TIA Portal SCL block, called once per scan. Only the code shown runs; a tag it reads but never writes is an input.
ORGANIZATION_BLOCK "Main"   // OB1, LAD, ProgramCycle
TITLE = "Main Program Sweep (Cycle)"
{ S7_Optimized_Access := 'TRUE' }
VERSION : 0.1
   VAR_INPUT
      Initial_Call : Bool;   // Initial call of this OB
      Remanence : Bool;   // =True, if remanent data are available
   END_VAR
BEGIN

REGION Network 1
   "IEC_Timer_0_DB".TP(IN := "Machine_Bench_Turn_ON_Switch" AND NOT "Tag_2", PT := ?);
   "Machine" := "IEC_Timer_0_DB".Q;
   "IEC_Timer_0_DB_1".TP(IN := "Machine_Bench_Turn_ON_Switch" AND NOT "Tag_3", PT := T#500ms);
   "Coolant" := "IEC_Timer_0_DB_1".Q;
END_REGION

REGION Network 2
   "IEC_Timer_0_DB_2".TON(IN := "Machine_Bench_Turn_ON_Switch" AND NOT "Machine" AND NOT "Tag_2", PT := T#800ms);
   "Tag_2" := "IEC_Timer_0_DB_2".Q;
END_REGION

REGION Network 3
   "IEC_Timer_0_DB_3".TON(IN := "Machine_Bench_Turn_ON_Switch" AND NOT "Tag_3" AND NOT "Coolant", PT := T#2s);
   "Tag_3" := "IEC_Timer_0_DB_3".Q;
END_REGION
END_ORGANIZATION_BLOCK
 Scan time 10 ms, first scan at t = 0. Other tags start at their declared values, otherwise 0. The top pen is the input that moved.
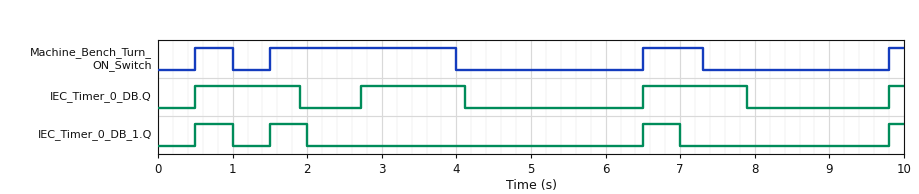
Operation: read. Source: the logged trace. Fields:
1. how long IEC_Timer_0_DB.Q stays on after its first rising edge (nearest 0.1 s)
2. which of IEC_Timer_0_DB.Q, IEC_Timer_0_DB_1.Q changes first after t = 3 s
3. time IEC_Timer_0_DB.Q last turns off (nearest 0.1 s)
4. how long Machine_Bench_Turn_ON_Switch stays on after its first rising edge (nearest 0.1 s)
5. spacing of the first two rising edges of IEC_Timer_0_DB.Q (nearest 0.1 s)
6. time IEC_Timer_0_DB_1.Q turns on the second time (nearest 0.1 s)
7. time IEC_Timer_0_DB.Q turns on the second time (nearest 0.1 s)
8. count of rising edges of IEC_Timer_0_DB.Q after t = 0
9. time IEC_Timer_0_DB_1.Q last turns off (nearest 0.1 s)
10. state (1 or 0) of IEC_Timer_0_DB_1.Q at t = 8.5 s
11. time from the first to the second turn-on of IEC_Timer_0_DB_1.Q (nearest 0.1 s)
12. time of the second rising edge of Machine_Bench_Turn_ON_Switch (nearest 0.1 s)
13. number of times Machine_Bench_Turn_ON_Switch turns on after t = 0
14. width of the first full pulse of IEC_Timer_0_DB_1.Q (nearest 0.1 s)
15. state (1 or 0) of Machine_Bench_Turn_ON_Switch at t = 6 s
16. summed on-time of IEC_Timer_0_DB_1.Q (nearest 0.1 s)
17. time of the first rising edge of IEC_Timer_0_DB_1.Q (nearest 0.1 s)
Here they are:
1.4 s
IEC_Timer_0_DB.Q
7.9 s
0.5 s
2.2 s
1.5 s
2.7 s
4
7.0 s
0
1.0 s
1.5 s
4
0.5 s
0
1.7 s
0.5 s
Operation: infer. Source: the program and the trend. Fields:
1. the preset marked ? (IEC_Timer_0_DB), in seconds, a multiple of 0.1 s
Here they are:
1.4 s
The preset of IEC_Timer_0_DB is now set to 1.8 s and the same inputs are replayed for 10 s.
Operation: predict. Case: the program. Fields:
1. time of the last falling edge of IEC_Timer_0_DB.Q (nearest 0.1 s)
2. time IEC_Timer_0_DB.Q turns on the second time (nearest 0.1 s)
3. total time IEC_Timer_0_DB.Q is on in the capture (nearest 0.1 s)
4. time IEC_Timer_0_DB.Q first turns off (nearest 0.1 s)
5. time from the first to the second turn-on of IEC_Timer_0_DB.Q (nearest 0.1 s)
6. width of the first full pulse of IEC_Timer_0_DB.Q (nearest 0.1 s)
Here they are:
8.3 s
3.1 s
5.6 s
2.3 s
2.6 s
1.8 s
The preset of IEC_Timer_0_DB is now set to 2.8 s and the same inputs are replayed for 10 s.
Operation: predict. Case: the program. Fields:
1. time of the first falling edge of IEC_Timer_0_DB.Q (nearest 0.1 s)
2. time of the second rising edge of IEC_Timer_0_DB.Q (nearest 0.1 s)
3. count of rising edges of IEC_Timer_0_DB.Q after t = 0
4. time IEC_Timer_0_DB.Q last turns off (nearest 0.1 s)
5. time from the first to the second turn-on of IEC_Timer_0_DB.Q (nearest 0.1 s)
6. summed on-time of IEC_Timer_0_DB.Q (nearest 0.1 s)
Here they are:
3.3 s
6.5 s
3
9.3 s
6.0 s
5.8 s
